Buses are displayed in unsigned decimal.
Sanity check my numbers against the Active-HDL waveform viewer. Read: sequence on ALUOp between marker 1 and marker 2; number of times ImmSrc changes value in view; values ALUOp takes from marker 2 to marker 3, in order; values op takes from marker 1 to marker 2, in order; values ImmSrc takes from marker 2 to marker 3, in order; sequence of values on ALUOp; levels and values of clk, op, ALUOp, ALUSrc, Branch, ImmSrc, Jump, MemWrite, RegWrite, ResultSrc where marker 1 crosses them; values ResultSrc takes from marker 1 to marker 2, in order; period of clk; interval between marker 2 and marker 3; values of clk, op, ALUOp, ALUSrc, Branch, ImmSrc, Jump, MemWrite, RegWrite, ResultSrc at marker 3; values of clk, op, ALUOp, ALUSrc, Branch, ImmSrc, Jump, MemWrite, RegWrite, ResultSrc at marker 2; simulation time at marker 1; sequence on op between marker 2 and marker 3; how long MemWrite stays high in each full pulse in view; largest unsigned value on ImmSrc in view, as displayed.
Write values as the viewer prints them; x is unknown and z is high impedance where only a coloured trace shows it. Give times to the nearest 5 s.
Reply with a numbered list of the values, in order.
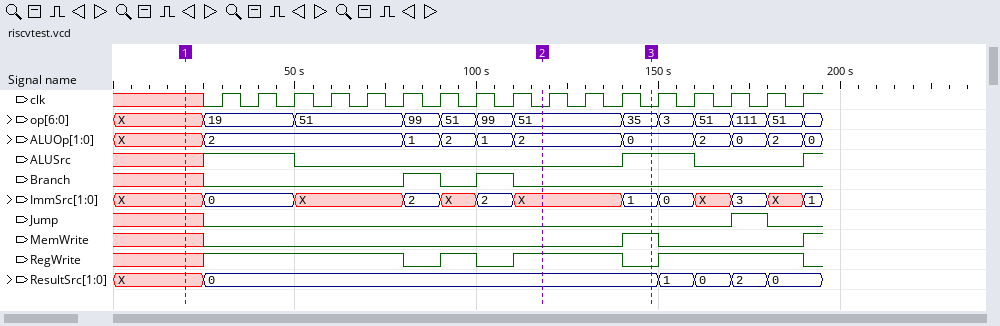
1. X, 2, 1, 2, 1, 2
2. 12
3. 2, 0
4. X, 19, 51, 99, 51, 99, 51
5. X, 1
6. X, 2, 1, 2, 1, 2, 0, 2, 0, 2, 0
7. clk=x, op=X, ALUOp=X, ALUSrc=x, Branch=x, ImmSrc=X, Jump=x, MemWrite=x, RegWrite=x, ResultSrc=X
8. X, 0
9. 10 s
10. 30 s
11. clk=0, op=35, ALUOp=0, ALUSrc=1, Branch=0, ImmSrc=1, Jump=0, MemWrite=1, RegWrite=0, ResultSrc=0
12. clk=0, op=51, ALUOp=2, ALUSrc=0, Branch=0, ImmSrc=X, Jump=0, MemWrite=0, RegWrite=1, ResultSrc=0
13. 20 s
14. 51, 35
15. 10 s
16. 3
